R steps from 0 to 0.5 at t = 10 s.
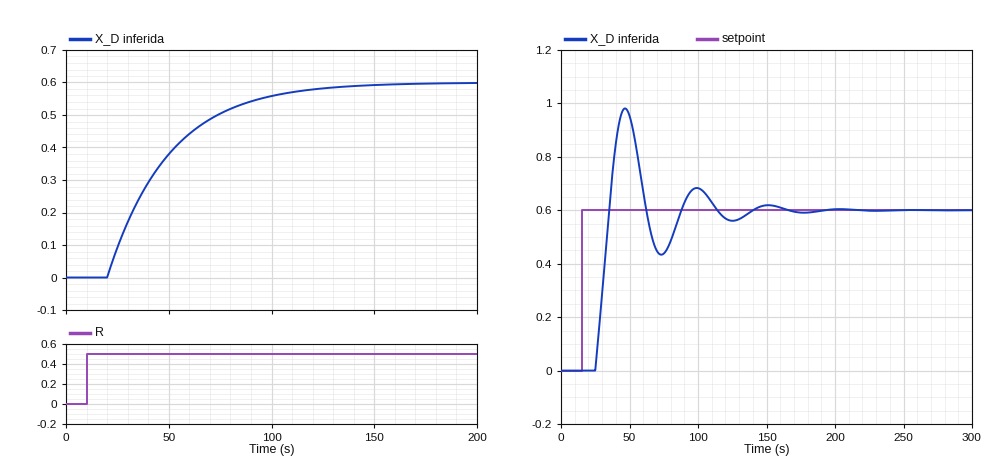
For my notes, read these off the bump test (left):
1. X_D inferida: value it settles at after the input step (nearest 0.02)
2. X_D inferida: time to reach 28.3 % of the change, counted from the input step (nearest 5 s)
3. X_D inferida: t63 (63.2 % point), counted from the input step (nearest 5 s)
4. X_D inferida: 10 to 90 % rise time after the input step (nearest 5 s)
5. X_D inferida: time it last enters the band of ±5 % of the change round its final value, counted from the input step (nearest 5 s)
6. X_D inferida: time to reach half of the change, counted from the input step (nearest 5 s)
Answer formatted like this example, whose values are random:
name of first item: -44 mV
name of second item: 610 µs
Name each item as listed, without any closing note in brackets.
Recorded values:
X_D inferida: value it settles at after the input step: 0.60
X_D inferida: time to reach 28.3 % of the change, counted from the input step: 20 s
X_D inferida: t63 (63.2 % point), counted from the input step: 40 s
X_D inferida: 10 to 90 % rise time after the input step: 65 s
X_D inferida: time it last enters the band of ±5 % of the change round its final value, counted from the input step: 100 s
X_D inferida: time to reach half of the change, counted from the input step: 30 s
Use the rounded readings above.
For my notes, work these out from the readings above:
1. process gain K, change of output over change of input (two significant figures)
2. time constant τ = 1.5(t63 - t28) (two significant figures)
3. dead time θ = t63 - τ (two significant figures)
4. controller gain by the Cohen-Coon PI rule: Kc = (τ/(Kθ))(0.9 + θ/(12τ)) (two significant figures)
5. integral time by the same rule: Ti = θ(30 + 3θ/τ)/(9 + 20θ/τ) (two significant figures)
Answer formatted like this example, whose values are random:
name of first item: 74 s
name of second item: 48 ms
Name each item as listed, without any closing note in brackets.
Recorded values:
process gain K, change of output over change of input: 1.2
time constant τ = 1.5(t63 - t28): 30 s
dead time θ = t63 - τ: 10 s
controller gain by the Cohen-Coon PI rule: Kc = (τ/(Kθ))(0.9 + θ/(12τ)): 2.3
integral time by the same rule: Ti = θ(30 + 3θ/τ)/(9 + 20θ/τ): 20 s
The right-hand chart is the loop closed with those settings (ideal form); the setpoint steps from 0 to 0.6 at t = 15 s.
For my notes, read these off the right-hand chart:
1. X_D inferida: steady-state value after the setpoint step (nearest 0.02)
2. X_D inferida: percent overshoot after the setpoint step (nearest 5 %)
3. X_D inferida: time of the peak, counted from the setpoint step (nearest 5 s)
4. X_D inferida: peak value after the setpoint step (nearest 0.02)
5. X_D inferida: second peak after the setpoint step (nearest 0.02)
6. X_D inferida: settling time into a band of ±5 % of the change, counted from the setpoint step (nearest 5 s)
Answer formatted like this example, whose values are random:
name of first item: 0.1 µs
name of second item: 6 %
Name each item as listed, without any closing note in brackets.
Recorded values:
X_D inferida: steady-state value after the setpoint step: 0.60
X_D inferida: percent overshoot after the setpoint step: 65 %
X_D inferida: time of the peak, counted from the setpoint step: 30 s
X_D inferida: peak value after the setpoint step: 0.98
X_D inferida: second peak after the setpoint step: 0.68
X_D inferida: settling time into a band of ±5 % of the change, counted from the setpoint step: 115 s
